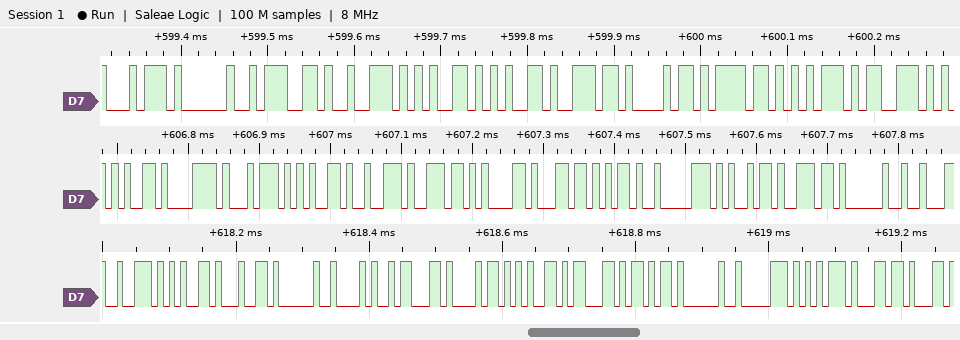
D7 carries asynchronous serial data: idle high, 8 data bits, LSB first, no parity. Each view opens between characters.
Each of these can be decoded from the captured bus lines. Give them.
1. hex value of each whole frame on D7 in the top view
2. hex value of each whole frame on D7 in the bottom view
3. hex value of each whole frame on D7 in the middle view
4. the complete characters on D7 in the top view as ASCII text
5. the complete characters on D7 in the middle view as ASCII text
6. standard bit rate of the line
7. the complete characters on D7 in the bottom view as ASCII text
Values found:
74, 20, 67, 72, 65, 65, 6E, 68, 6F, 75, 73
72, 65, 64, 20, 28, 63, 68, 65, 63, 6B, 20, 70, 75, 6C
65, 78, 74, 65, 72, 6E, 61, 6C, 2D, 70, 69, 6E, 20
"t greenhous"
"external-pin "
115200 baud
"red (check pul"
